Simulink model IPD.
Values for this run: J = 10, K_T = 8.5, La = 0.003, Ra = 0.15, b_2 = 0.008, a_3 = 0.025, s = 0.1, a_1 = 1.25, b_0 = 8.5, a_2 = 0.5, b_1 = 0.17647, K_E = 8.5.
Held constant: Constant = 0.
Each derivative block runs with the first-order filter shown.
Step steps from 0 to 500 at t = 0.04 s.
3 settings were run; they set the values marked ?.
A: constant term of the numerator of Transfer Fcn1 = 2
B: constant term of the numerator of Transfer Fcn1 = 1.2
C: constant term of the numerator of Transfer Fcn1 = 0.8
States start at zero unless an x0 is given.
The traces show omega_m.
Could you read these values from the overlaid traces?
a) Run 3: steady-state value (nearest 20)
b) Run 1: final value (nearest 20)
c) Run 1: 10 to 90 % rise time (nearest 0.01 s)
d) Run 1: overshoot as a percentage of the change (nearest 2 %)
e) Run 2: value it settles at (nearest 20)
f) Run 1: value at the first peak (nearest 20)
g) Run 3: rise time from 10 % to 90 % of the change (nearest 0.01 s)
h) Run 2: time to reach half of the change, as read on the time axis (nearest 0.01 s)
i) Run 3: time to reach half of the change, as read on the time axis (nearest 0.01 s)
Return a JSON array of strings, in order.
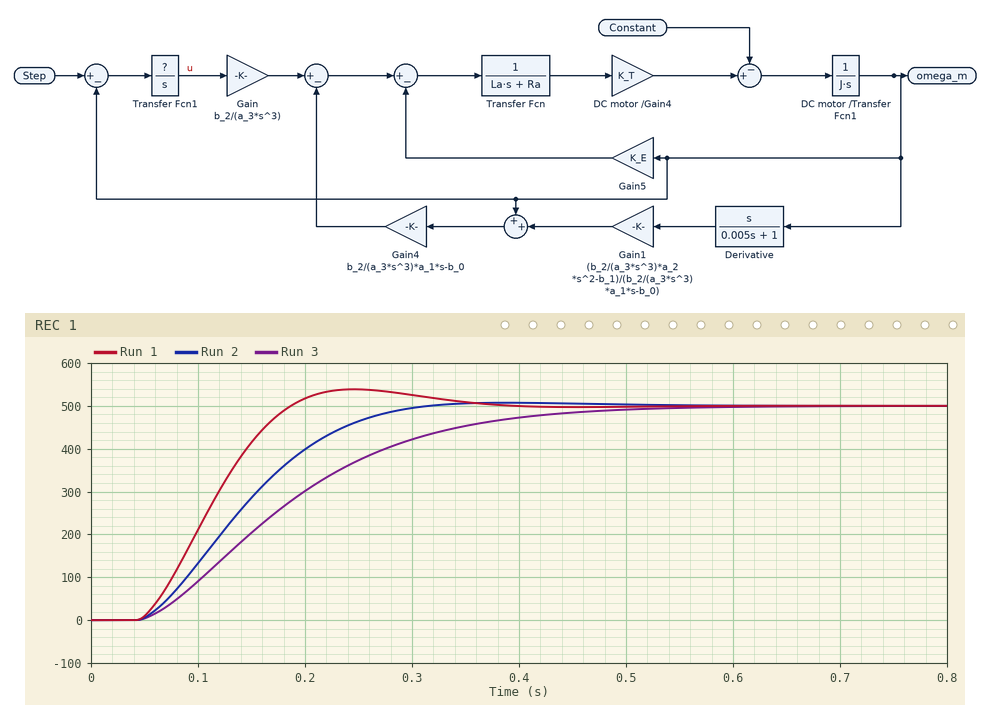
["500", "500", "0.10 s", "8 %", "500", "540", "0.26 s", "0.14 s", "0.17 s"]
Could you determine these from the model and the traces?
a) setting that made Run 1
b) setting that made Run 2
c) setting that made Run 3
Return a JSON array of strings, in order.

["A", "B", "C"]
